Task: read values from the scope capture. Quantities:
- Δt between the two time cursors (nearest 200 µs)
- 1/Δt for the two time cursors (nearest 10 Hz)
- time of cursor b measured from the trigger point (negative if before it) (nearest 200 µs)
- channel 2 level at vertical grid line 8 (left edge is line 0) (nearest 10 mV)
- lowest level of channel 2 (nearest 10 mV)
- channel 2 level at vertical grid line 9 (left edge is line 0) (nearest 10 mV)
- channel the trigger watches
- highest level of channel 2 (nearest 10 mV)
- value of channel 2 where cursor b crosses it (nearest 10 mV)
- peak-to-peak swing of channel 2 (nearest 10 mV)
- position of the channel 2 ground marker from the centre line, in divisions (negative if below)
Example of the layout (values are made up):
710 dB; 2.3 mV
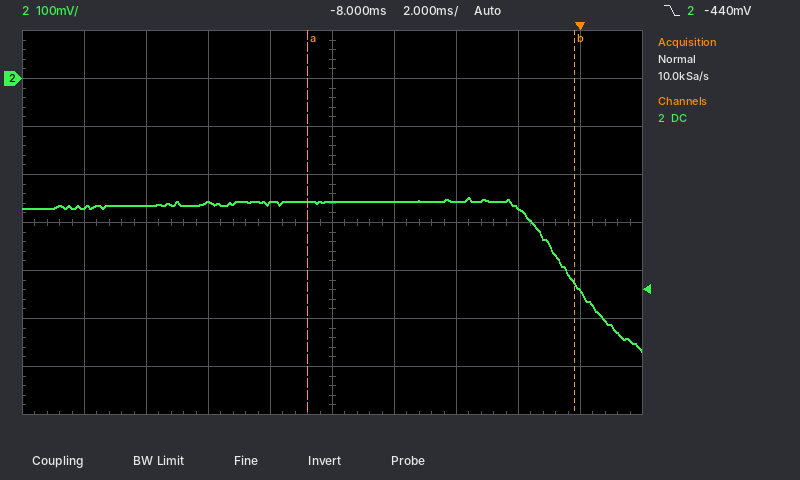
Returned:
8.6 ms; 120 Hz; -200 µs; -270 mV; -570 mV; -440 mV; channel 2; -250 mV; -430 mV; 320 mV; +3.0 div
